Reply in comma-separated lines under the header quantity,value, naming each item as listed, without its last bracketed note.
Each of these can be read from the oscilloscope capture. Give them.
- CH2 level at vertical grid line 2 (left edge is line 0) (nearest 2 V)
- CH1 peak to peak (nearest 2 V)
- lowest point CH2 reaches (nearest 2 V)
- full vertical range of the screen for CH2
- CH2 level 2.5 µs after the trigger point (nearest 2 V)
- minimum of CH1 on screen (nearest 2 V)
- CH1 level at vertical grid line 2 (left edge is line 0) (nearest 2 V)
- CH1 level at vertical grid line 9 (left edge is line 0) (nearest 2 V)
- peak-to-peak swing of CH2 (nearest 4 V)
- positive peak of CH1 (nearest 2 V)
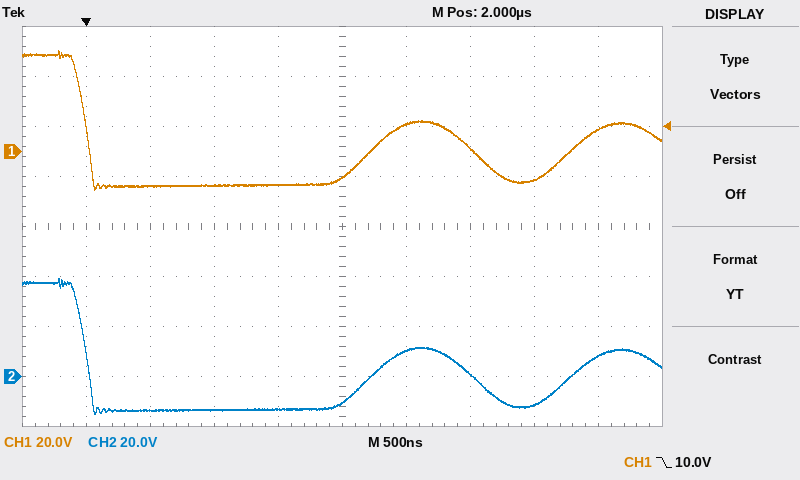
quantity,value
CH2 level at vertical grid line 2 (left edge is line 0),-14 V
CH1 peak to peak,56 V
lowest point CH2 reaches,-16 V
full vertical range of the screen for CH2,160 V
CH2 level 2.5 µs after the trigger point,10 V
minimum of CH1 on screen,-16 V
CH1 level at vertical grid line 2 (left edge is line 0),-14 V
CH1 level at vertical grid line 9 (left edge is line 0),8 V
peak-to-peak swing of CH2,56 V
positive peak of CH1,40 V
